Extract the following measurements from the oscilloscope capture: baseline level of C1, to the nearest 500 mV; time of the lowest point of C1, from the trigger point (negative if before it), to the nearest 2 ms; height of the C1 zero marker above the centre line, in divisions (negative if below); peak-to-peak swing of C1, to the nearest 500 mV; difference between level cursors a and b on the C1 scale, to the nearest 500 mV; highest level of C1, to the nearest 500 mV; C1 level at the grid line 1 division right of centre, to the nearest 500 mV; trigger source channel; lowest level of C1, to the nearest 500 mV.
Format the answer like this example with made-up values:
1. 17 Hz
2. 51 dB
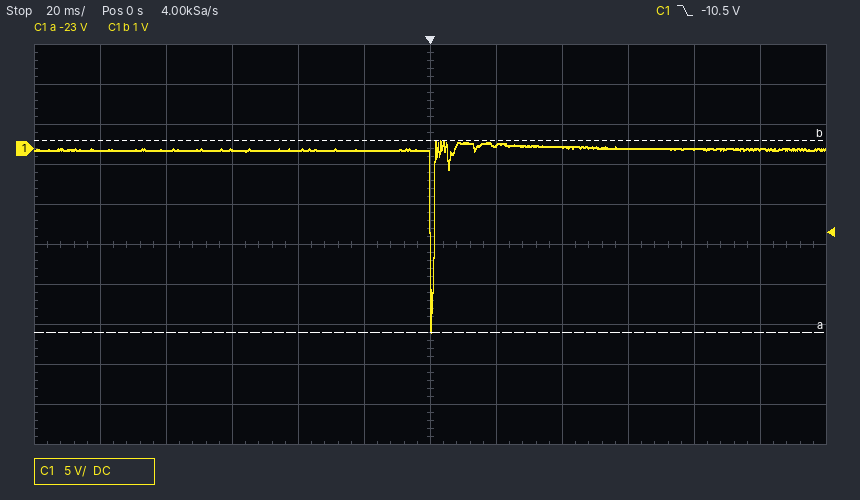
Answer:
1. 0.0 V
2. 0 ms
3. +2.4 div
4. 24.0 V
5. 24.0 V
6. 1.0 V
7. 500 mV
8. C1
9. -23.0 V
